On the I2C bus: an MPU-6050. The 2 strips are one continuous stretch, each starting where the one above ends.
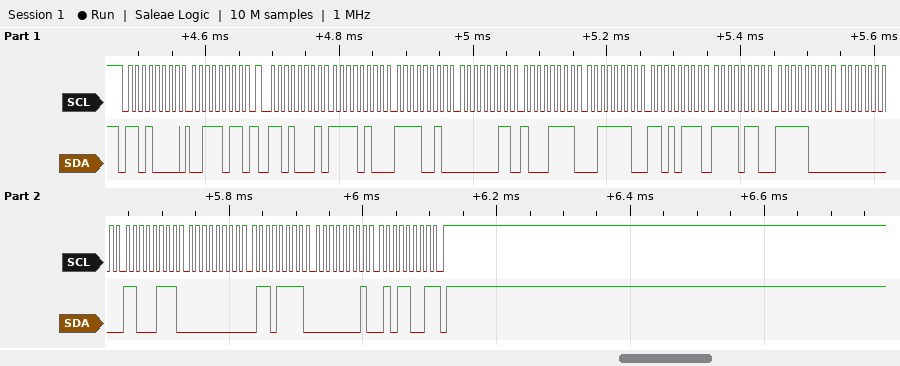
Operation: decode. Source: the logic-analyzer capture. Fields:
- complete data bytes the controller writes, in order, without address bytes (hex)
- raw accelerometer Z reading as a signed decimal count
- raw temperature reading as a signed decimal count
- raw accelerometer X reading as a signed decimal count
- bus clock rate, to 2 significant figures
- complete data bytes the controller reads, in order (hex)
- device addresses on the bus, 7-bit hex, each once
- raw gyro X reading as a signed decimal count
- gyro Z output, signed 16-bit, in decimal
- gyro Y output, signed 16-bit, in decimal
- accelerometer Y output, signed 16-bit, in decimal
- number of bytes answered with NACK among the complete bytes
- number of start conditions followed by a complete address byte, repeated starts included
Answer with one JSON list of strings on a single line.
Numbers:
["3B", "16087", "-2312", "-2830", "100 kHz", "F4 F2 03 8F 3E D7 F6 F8 00 C7 00 6F 01 59", "0x68", "199", "345", "111", "911", "1", "2"]
